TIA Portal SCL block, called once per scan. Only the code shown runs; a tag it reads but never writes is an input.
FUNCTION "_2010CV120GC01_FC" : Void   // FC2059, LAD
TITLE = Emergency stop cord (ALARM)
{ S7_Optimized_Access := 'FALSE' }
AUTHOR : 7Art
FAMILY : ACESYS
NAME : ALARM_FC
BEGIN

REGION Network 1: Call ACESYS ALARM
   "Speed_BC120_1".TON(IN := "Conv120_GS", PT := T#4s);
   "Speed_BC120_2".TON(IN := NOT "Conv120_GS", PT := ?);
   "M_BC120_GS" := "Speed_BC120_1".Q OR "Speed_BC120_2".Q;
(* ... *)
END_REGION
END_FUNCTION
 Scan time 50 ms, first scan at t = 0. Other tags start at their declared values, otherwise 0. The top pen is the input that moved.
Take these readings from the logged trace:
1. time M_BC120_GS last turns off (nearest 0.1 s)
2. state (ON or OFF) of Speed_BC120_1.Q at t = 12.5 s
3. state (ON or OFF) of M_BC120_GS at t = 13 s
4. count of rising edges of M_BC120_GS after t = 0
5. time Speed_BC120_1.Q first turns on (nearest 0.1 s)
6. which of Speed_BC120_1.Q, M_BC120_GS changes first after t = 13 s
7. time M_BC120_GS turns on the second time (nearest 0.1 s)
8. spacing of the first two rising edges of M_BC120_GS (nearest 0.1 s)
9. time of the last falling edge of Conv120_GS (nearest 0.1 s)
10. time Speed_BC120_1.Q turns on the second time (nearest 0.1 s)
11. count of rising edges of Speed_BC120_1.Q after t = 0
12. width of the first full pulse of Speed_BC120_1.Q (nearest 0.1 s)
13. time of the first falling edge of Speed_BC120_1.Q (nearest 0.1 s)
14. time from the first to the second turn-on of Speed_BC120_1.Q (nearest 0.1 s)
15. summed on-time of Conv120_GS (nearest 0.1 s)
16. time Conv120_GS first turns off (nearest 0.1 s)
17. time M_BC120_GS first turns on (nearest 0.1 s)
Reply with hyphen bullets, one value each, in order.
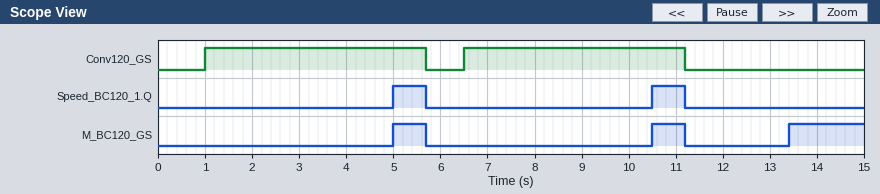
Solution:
- 11.2 s
- OFF
- OFF
- 3
- 5.0 s
- M_BC120_GS
- 10.5 s
- 5.5 s
- 11.2 s
- 10.5 s
- 2
- 0.7 s
- 5.7 s
- 5.5 s
- 9.4 s
- 5.7 s
- 5.0 s
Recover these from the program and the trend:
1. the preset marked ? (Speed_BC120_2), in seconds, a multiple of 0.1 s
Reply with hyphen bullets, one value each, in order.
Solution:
- 2.2 s
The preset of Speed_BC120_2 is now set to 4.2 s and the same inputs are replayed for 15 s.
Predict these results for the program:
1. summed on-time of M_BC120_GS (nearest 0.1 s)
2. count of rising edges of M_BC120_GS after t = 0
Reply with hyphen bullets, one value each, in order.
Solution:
- 1.4 s
- 2
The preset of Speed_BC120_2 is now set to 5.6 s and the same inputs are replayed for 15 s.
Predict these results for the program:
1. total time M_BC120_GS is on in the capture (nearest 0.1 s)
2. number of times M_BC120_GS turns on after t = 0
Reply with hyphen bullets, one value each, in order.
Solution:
- 1.4 s
- 2
